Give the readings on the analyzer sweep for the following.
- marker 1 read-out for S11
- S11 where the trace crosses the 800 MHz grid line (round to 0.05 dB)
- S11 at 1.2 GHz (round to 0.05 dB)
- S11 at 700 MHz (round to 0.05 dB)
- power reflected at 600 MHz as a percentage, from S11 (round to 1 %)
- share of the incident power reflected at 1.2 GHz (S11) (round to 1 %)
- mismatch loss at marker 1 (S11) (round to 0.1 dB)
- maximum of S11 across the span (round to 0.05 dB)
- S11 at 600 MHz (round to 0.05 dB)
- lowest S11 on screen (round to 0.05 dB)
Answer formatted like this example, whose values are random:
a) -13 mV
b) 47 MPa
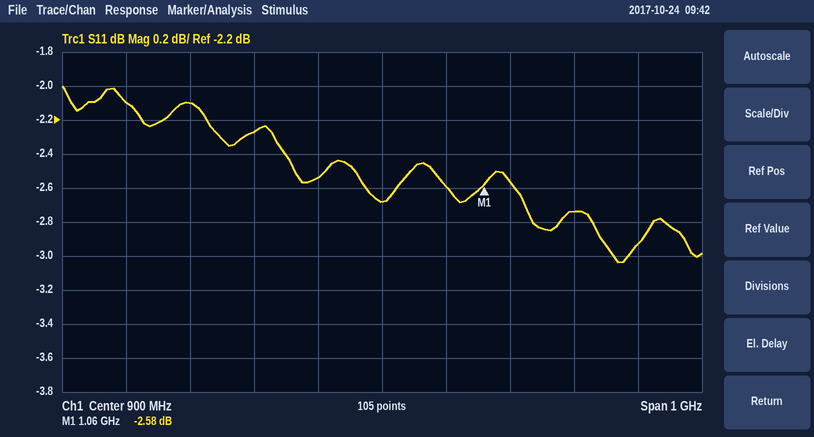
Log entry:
a) -2.58 dB
b) -2.55 dB
c) -2.75 dB
d) -2.25 dB
e) 62 %
f) 53 %
g) 3.5 dB
h) -2.00 dB
i) -2.10 dB
j) -3.05 dB
